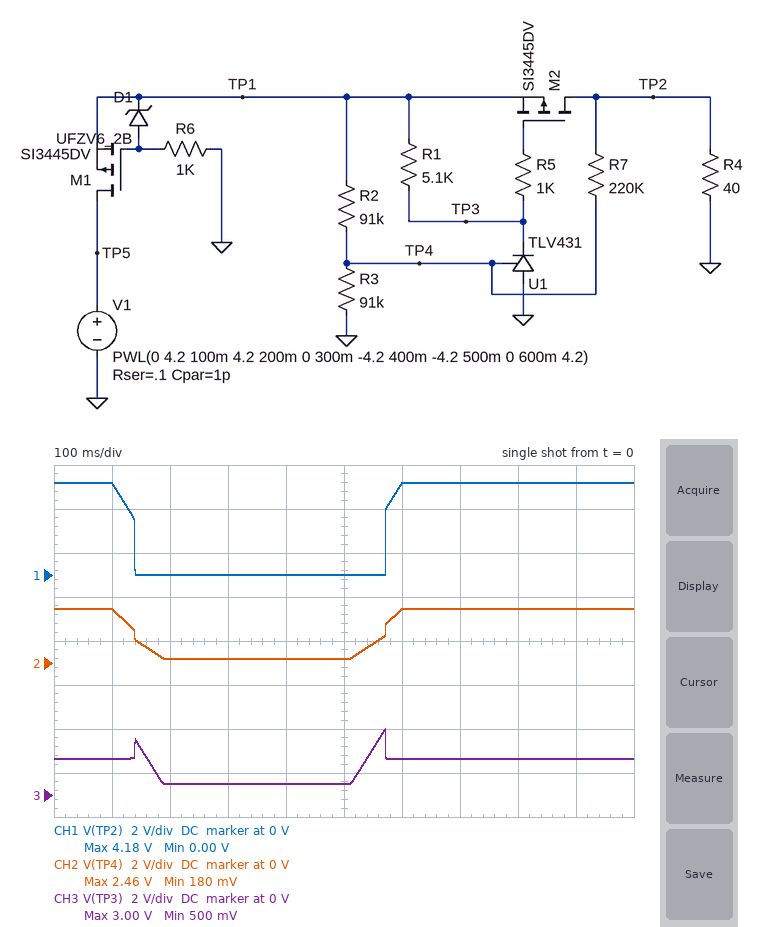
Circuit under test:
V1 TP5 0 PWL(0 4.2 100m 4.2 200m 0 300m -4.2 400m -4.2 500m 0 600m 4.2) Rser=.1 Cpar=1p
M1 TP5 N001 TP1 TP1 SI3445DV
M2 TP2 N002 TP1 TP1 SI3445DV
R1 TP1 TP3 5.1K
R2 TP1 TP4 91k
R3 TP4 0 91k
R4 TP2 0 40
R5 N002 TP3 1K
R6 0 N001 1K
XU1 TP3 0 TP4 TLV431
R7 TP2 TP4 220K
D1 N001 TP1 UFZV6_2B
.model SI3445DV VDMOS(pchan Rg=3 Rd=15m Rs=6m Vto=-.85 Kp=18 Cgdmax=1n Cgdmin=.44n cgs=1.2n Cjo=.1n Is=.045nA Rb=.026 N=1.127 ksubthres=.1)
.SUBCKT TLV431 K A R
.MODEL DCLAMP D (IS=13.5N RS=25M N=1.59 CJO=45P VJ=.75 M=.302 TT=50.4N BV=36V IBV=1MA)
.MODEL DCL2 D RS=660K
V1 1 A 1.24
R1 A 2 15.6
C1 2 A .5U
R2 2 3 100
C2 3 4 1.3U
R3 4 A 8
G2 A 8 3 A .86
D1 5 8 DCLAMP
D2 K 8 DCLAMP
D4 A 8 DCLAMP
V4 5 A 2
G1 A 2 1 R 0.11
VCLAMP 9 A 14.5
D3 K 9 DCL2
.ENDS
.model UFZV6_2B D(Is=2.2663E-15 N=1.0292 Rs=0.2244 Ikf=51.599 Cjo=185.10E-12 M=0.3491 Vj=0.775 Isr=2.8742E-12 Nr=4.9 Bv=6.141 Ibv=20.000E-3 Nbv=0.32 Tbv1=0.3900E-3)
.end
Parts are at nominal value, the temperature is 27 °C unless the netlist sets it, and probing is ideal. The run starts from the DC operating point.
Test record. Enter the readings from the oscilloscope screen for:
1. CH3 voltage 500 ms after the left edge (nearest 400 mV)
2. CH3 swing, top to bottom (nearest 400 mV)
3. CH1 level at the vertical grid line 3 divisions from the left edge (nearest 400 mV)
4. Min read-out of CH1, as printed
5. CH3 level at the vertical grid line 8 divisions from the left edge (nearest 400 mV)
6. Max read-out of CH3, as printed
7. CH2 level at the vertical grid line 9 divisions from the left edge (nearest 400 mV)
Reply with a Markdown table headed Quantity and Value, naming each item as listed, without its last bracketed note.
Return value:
| Quantity | Value |
|---|---|
| CH3 voltage 500 ms after the left edge | 400 mV |
| CH3 swing, top to bottom | 2.4 V |
| CH1 level at the vertical grid line 3 divisions from the left edge | 0 V |
| Min read-out of CH1, as printed | 0.00 V |
| CH3 level at the vertical grid line 8 divisions from the left edge | 1.6 V |
| Max read-out of CH3, as printed | 3.00 V |
| CH2 level at the vertical grid line 9 divisions from the left edge | 2.4 V |
